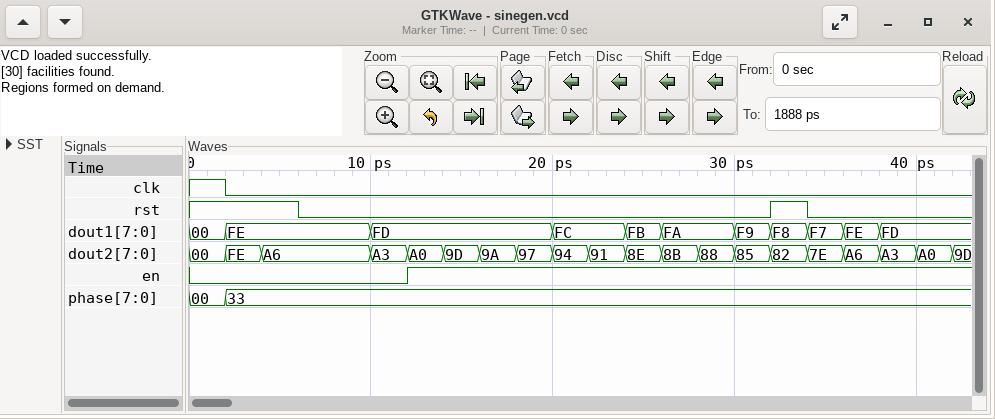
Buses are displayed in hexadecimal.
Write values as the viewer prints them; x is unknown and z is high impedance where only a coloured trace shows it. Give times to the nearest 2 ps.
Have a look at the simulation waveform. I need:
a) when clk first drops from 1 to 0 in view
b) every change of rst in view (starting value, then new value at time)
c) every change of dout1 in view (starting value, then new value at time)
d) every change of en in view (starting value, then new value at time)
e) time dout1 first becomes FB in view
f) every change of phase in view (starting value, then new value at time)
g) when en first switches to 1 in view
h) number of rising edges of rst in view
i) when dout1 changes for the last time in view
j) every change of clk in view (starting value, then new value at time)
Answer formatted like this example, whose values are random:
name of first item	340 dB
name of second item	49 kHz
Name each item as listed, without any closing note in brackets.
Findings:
when clk first drops from 1 to 0 in view	2 ps
every change of rst in view	1, 0 at 6 ps, 1 at 32 ps, 0 at 34 ps
every change of dout1 in view	00, FE at 2 ps, FD at 10 ps, FC at 20 ps, FB at 24 ps, FA at 26 ps, F9 at 30 ps, F8 at 32 ps, F7 at 34 ps, FE at 36 ps, FD at 38 ps
every change of en in view	0, 1 at 12 ps
time dout1 first becomes FB in view	24 ps
every change of phase in view	00, 33 at 2 ps
when en first switches to 1 in view	12 ps
number of rising edges of rst in view	1
when dout1 changes for the last time in view	38 ps
every change of clk in view	1, 0 at 2 ps
